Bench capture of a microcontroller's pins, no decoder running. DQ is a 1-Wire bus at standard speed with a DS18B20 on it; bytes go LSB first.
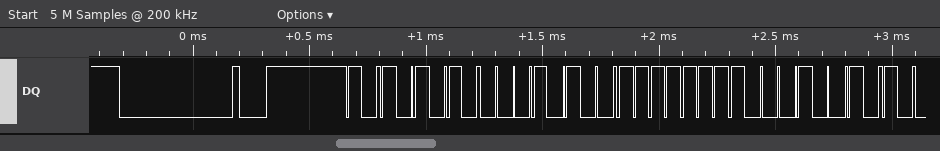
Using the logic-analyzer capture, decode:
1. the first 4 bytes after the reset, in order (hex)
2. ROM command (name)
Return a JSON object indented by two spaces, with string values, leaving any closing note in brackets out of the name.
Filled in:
{
  "the first 4 bytes after the reset, in order": "55 28 FF 48",
  "ROM command": "Match ROM"
}
